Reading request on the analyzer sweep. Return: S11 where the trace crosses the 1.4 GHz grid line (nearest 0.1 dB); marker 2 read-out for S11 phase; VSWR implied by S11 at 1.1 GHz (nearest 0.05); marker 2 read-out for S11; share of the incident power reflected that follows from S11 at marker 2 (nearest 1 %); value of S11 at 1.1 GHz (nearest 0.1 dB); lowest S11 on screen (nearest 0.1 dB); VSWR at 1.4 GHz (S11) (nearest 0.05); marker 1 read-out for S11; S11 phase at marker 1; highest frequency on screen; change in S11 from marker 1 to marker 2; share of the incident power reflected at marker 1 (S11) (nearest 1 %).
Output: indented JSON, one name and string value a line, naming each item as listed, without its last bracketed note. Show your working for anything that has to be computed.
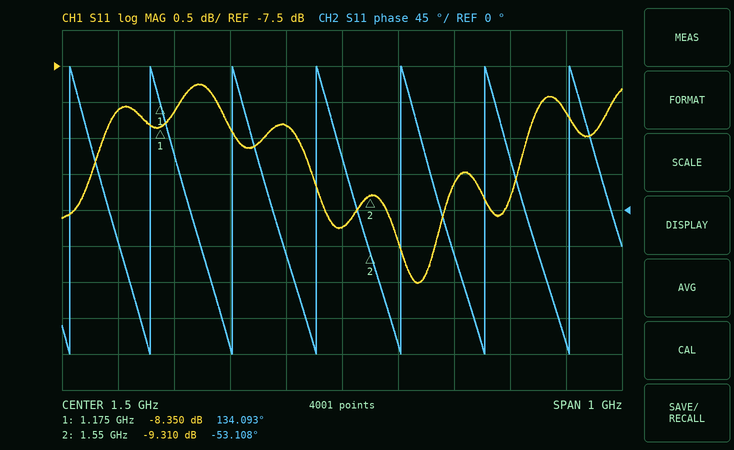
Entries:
{
  "S11 where the trace crosses the 1.4 GHz grid line": "-8.3 dB",
  "marker 2 read-out for S11 phase": "-53.108°",
  "VSWR implied by S11 at 1.1 GHz": "|Γ| = 10^(-8.1/20) = 0.3936; VSWR = (1 + 0.3936)/(1 − 0.3936) ≈ 2.30",
  "marker 2 read-out for S11": "-9.310 dB",
  "share of the incident power reflected that follows from S11 at marker 2": "10^(-9.31/10) ≈ 12 %",
  "value of S11 at 1.1 GHz": "-8.1 dB",
  "lowest S11 on screen": "-10.5 dB",
  "VSWR at 1.4 GHz (S11)": "|Γ| = 10^(-8.3/20) = 0.3846; VSWR = (1 + 0.3846)/(1 − 0.3846) ≈ 2.25",
  "marker 1 read-out for S11": "-8.350 dB",
  "S11 phase at marker 1": "134.093°",
  "highest frequency on screen": "2 GHz",
  "change in S11 from marker 1 to marker 2": "-9.31 − (-8.35) = -0.960 dB",
  "share of the incident power reflected at marker 1 (S11)": "10^(-8.35/10) ≈ 15 %"
}
